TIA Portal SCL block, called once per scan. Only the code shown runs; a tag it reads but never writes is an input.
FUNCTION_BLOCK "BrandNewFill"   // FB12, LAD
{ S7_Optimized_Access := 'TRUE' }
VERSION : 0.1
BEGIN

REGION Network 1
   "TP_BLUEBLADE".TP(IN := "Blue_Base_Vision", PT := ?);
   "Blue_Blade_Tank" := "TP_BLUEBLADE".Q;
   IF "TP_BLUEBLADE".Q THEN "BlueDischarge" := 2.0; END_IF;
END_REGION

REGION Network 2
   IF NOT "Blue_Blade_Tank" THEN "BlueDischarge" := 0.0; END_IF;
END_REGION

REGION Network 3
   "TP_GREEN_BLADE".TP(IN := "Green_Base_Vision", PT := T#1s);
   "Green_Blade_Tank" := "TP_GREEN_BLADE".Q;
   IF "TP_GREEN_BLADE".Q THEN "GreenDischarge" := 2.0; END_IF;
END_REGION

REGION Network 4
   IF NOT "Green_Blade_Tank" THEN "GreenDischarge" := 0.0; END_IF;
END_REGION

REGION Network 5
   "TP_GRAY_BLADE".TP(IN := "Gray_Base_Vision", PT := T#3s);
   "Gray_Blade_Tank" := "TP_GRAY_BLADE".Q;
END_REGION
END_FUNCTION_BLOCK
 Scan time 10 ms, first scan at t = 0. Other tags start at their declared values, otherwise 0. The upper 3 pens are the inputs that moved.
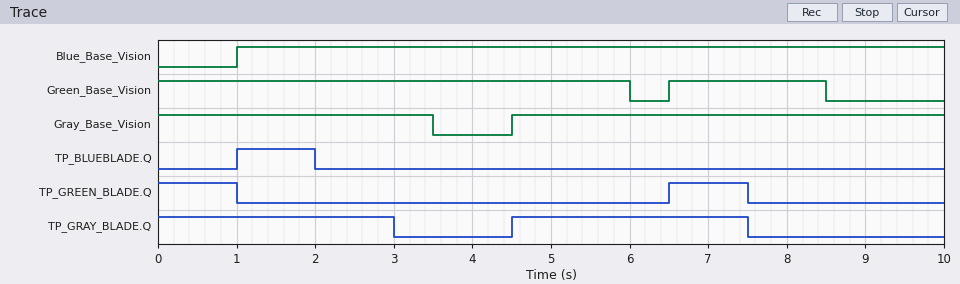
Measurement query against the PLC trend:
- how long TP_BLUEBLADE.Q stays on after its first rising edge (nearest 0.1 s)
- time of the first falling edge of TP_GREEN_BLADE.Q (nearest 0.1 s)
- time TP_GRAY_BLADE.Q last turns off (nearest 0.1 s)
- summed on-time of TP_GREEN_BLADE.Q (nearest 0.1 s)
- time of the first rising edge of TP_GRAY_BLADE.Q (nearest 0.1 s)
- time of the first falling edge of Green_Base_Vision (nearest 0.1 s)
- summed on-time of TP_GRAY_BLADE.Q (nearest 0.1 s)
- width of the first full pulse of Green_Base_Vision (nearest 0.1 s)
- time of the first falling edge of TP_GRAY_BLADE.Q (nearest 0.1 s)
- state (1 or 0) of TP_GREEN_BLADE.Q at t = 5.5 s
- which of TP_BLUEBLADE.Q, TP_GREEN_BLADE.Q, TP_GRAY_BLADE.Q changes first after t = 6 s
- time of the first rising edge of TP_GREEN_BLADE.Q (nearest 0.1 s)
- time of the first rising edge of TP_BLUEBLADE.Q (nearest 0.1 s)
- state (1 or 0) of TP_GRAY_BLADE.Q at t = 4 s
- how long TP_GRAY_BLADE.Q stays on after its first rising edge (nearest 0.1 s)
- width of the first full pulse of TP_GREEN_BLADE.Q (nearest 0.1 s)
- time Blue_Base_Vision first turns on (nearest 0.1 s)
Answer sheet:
1.0 s
1.0 s
7.5 s
2.0 s
4.5 s
6.0 s
6.0 s
2.0 s
3.0 s
0
TP_GREEN_BLADE.Q
6.5 s
1.0 s
0
3.0 s
1.0 s
1.0 s
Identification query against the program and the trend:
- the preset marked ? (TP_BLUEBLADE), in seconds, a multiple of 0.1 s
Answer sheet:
1.0 s
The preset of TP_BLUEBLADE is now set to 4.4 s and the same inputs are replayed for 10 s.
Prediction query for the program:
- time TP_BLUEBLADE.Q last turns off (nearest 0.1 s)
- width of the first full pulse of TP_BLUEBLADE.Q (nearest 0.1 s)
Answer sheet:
5.4 s
4.4 s
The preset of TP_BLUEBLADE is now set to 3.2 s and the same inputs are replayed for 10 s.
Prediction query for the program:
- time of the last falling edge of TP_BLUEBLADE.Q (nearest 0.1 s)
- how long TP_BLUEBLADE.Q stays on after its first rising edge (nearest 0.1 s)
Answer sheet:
4.2 s
3.2 s
